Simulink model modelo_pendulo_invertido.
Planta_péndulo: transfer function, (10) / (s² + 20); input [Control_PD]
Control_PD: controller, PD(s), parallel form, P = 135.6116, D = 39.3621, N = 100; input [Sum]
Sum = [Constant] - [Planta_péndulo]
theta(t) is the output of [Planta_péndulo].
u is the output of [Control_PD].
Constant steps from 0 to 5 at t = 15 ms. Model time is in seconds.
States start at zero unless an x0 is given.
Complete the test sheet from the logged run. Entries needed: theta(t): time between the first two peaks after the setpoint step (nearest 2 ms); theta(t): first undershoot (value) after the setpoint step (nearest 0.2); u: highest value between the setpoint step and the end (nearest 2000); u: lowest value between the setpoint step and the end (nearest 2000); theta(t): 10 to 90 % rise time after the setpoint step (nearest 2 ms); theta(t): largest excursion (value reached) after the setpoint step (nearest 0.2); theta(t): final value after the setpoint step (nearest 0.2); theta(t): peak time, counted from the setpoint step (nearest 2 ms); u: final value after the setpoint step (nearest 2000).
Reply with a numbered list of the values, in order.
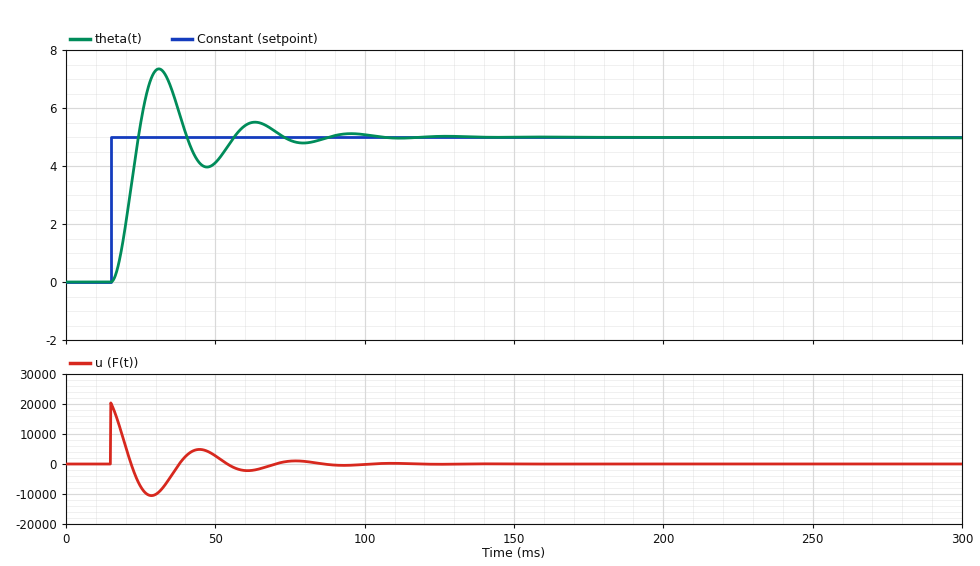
1. 32 ms
2. 4.0
3. 20000
4. -10000
5. 6 ms
6. 7.4
7. 5.0
8. 16 ms
9. 0
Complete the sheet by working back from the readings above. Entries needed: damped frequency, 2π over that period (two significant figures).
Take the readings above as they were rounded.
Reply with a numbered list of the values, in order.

1. 0.20 rad/ms
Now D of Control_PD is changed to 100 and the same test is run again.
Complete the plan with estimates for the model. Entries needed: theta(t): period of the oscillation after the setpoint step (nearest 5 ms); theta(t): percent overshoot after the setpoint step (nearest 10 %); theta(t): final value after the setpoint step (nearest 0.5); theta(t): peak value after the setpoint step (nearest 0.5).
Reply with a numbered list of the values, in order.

1. 20 ms
2. 60 %
3. 5.0
4. 8.0
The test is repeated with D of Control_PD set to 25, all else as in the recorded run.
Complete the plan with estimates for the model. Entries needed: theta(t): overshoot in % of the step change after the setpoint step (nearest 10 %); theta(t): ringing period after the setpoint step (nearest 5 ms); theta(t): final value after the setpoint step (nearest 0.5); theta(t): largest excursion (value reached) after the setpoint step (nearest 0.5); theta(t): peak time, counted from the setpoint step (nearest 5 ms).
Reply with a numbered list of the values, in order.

1. 40 %
2. 40 ms
3. 5.0
4. 7.0
5. 20 ms
